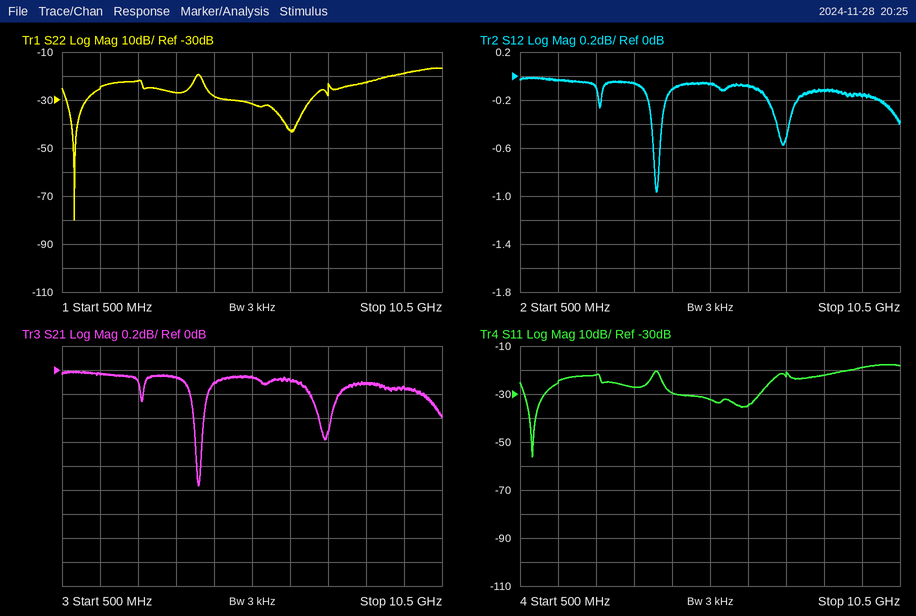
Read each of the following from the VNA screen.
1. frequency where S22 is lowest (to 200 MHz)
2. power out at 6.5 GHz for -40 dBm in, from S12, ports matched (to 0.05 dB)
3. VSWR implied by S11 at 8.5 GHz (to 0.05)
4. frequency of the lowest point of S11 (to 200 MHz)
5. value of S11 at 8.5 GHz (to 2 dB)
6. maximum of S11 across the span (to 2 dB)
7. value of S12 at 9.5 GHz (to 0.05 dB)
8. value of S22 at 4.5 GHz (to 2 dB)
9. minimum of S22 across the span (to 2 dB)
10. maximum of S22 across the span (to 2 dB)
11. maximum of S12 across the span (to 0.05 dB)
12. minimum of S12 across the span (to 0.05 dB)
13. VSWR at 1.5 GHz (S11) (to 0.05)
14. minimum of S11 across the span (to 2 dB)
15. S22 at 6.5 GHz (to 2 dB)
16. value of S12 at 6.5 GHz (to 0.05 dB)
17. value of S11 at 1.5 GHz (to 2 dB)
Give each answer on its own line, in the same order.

800 MHz
-40.10 dBm
1.15
800 MHz
-22 dB
-18 dB
-0.15 dB
-28 dB
-80 dB
-16 dB
0.00 dB
-0.95 dB
1.10
-56 dB
-42 dB
-0.10 dB
-26 dB
